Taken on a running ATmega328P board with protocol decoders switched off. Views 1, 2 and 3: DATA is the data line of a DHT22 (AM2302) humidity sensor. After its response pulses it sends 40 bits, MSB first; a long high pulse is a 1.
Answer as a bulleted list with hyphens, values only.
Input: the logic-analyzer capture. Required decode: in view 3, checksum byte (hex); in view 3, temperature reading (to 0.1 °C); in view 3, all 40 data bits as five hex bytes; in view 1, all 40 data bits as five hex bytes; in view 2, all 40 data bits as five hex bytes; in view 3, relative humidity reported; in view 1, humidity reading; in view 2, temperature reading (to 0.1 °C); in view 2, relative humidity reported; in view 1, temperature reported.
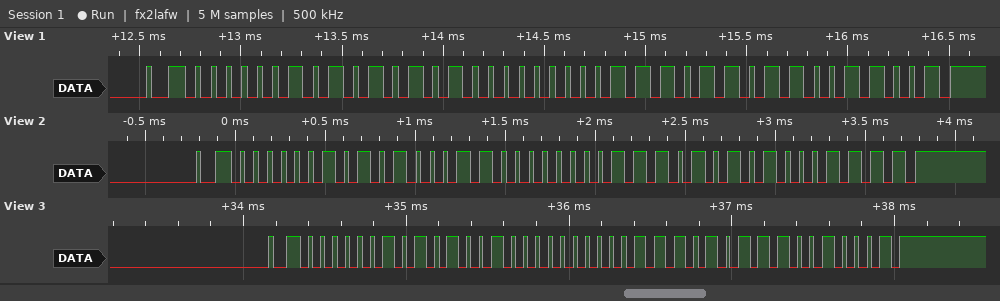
- 0x91
- 23.5 °C
- 02 A4 00 EB 91
- 02 AA 00 ED 99
- 02 A3 00 EA 8F
- 67.6 %
- 68.2 %
- 23.4 °C
- 67.5 %
- 23.7 °C
